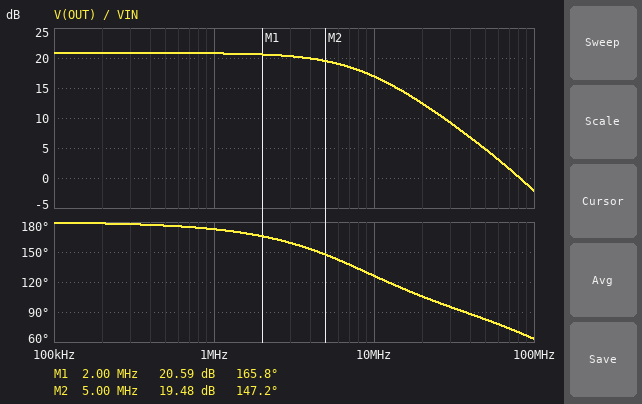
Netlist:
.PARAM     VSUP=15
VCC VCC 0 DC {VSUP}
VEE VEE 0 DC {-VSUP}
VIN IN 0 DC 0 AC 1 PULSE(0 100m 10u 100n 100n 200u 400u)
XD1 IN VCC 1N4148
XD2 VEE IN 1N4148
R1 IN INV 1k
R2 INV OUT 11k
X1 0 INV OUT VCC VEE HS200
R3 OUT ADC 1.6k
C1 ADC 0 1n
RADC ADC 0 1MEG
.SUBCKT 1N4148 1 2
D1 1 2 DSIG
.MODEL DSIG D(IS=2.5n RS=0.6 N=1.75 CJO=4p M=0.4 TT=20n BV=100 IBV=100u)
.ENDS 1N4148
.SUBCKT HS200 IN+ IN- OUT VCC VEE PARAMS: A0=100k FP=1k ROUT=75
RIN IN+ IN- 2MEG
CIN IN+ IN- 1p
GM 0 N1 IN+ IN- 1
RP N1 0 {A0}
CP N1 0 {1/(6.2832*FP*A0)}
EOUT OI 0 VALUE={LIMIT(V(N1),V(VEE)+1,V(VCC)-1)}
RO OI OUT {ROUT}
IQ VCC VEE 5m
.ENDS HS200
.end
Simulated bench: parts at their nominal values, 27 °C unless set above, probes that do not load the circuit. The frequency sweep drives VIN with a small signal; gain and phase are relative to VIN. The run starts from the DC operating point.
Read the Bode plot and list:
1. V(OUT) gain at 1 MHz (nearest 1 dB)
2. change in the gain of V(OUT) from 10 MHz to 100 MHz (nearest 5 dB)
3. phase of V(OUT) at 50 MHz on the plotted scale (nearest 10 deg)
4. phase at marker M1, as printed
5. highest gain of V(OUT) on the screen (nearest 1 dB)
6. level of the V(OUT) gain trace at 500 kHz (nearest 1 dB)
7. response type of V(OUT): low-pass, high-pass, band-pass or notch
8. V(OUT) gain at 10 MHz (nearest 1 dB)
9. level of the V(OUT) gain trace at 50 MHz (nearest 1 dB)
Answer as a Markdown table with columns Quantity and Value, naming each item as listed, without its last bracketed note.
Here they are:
| Quantity | Value |
|---|---|
| V(OUT) gain at 1 MHz | 21 dB |
| change in the gain of V(OUT) from 10 MHz to 100 MHz | -20 dB |
| phase of V(OUT) at 50 MHz on the plotted scale | 80 deg |
| phase at marker M1, as printed | 165.8 deg |
| highest gain of V(OUT) on the screen | 21 dB |
| level of the V(OUT) gain trace at 500 kHz | 21 dB |
| response type of V(OUT): low-pass, high-pass, band-pass or notch | low-pass |
| V(OUT) gain at 10 MHz | 17 dB |
| level of the V(OUT) gain trace at 50 MHz | 5 dB |
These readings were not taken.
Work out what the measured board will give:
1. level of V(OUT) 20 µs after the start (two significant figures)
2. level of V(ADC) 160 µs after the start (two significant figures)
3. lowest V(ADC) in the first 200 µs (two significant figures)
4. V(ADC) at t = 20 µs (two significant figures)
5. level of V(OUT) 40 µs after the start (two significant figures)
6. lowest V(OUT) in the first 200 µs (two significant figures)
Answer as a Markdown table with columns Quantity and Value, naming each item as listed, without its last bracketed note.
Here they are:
| Quantity | Value |
|---|---|
| level of V(OUT) 20 µs after the start | -1.1 V |
| level of V(ADC) 160 µs after the start | -1.1 V |
| lowest V(ADC) in the first 200 µs | -1.1 V |
| V(ADC) at t = 20 µs | -1.1 V |
| level of V(OUT) 40 µs after the start | -1.1 V |
| lowest V(OUT) in the first 200 µs | -1.1 V |
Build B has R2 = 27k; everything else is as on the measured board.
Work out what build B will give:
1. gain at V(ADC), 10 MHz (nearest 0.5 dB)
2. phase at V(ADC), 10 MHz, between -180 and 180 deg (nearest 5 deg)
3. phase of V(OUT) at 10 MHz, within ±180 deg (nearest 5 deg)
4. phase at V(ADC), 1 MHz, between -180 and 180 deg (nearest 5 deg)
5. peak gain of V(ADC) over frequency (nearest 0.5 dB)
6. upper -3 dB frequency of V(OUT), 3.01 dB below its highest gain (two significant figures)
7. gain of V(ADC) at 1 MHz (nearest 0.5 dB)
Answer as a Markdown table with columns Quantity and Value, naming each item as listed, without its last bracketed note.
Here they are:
| Quantity | Value |
|---|---|
| gain at V(ADC), 10 MHz | -21.0 dB |
| phase at V(ADC), 10 MHz, between -180 and 180 deg | 15 deg |
| phase of V(OUT) at 10 MHz, within ±180 deg | 105 deg |
| phase at V(ADC), 1 MHz, between -180 and 180 deg | 80 deg |
| peak gain of V(ADC) over frequency | 28.5 dB |
| upper -3 dB frequency of V(OUT), 3.01 dB below its highest gain | 3.5 MHz |
| gain of V(ADC) at 1 MHz | 8.0 dB |
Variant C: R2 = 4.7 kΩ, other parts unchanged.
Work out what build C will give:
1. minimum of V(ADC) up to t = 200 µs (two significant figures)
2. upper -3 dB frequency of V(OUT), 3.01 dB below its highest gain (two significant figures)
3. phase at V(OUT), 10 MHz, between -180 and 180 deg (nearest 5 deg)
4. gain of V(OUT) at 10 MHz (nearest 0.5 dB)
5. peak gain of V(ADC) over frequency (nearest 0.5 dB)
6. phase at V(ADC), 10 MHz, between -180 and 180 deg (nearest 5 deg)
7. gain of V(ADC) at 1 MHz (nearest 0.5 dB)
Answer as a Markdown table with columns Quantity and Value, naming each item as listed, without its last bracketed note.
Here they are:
| Quantity | Value |
|---|---|
| minimum of V(ADC) up to t = 200 µs | -470 mV |
| upper -3 dB frequency of V(OUT), 3.01 dB below its highest gain | 18 MHz |
| phase at V(OUT), 10 MHz, between -180 and 180 deg | 150 deg |
| gain of V(OUT) at 10 MHz | 12.5 dB |
| peak gain of V(ADC) over frequency | 13.5 dB |
| phase at V(ADC), 10 MHz, between -180 and 180 deg | 60 deg |
| gain of V(ADC) at 1 MHz | -6.5 dB |
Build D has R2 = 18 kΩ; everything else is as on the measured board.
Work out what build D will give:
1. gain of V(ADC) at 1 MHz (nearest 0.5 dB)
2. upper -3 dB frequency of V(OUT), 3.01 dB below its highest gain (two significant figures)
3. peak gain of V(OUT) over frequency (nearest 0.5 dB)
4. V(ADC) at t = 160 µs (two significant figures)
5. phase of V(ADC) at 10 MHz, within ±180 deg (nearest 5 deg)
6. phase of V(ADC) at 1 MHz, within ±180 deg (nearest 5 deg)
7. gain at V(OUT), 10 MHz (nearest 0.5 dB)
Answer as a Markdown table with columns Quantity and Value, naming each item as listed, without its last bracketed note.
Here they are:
| Quantity | Value |
|---|---|
| gain of V(ADC) at 1 MHz | 5.0 dB |
| upper -3 dB frequency of V(OUT), 3.01 dB below its highest gain | 5.2 MHz |
| peak gain of V(OUT) over frequency | 25.0 dB |
| V(ADC) at t = 160 µs | -1.8 V |
| phase of V(ADC) at 10 MHz, within ±180 deg | 25 deg |
| phase of V(ADC) at 1 MHz, within ±180 deg | 85 deg |
| gain at V(OUT), 10 MHz | 18.5 dB |
